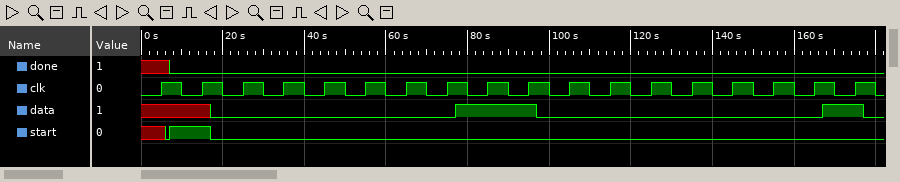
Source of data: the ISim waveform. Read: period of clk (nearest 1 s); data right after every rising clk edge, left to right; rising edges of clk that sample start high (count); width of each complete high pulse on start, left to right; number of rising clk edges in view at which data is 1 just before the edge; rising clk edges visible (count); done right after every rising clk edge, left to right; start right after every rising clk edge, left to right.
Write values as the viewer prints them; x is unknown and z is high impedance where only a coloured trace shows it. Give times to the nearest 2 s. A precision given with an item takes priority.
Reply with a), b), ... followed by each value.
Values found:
a) 10 s
b) x x 0 0 0 0 0 0 1 1 0 0 0 0 0 0 0 1
c) 1
d) 10 s
e) 3
f) 18
g) x 0 0 0 0 0 0 0 0 0 0 0 0 0 0 0 0 0
h) x 1 0 0 0 0 0 0 0 0 0 0 0 0 0 0 0 0
